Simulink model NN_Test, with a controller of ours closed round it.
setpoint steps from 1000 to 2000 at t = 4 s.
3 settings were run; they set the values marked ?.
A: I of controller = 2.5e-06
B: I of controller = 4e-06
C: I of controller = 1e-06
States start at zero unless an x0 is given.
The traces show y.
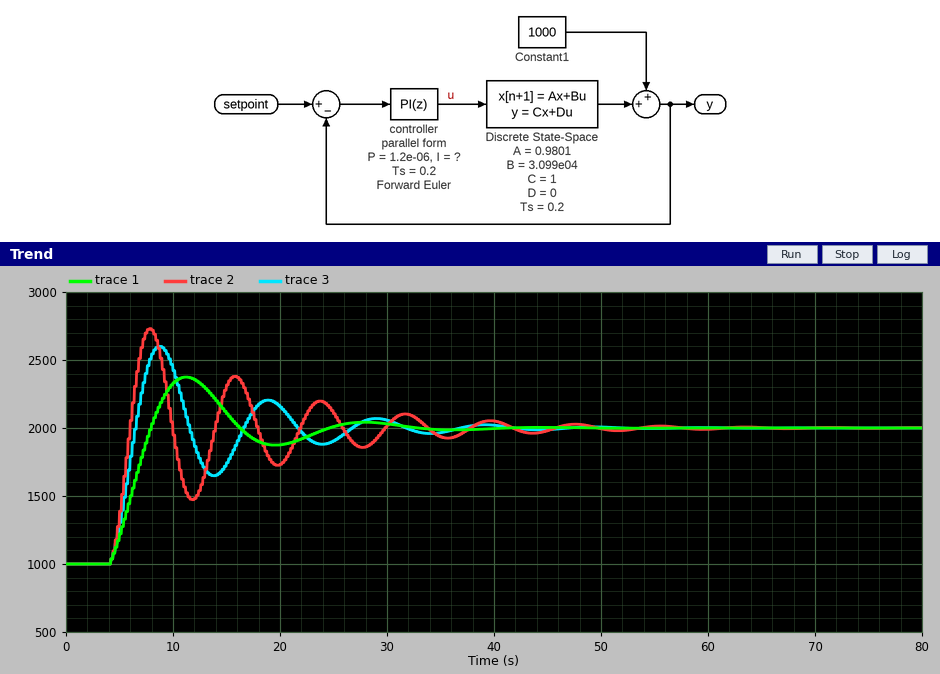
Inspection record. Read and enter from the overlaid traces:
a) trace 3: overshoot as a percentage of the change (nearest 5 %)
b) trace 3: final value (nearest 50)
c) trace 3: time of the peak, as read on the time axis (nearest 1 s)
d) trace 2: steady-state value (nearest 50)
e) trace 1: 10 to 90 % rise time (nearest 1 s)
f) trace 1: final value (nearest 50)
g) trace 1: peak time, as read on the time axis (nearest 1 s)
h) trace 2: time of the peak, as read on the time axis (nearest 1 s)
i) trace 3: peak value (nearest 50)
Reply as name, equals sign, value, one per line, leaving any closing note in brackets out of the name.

trace 3: overshoot as a percentage of the change = 60 %
trace 3: final value = 2000
trace 3: time of the peak, as read on the time axis = 9 s
trace 2: steady-state value = 2000
trace 1: 10 to 90 % rise time = 3 s
trace 1: final value = 2000
trace 1: peak time, as read on the time axis = 11 s
trace 2: time of the peak, as read on the time axis = 8 s
trace 3: peak value = 2600
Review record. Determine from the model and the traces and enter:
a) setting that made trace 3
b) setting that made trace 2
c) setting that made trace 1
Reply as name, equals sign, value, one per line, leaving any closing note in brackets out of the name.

setting that made trace 3 = A
setting that made trace 2 = B
setting that made trace 1 = C
